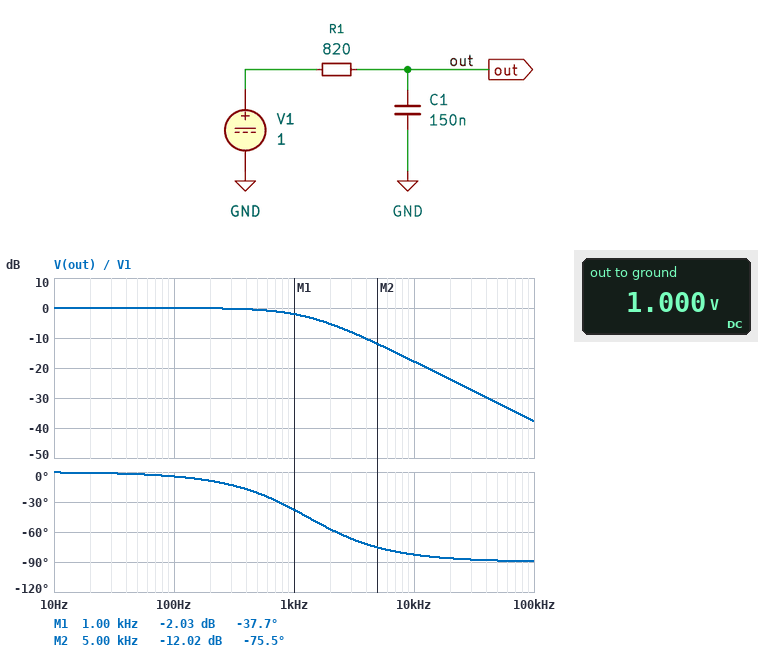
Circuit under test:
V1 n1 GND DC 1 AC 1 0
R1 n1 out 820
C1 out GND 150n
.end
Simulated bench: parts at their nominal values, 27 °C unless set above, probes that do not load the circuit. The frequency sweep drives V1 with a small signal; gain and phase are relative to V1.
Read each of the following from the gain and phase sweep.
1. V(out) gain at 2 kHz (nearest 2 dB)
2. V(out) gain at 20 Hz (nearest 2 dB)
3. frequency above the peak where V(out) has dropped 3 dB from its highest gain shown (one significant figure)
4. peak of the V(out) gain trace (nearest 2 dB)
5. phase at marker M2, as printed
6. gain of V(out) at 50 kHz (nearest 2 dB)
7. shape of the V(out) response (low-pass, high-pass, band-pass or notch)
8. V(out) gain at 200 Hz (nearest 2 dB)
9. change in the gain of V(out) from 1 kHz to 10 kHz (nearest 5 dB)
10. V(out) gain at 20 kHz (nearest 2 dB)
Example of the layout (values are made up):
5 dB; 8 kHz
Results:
-6 dB; 0 dB; 1 kHz; 0 dB; -75.5 deg; -32 dB; low-pass; 0 dB; -15 dB; -24 dB
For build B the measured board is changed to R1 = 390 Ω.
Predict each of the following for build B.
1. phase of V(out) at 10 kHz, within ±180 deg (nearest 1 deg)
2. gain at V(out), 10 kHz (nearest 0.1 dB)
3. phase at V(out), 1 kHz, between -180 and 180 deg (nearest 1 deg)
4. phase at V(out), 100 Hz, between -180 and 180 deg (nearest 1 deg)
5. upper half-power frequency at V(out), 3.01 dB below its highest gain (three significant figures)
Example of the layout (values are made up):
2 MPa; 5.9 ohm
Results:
-75 deg; -11.6 dB; -20 deg; -2 deg; 2.72 kHz
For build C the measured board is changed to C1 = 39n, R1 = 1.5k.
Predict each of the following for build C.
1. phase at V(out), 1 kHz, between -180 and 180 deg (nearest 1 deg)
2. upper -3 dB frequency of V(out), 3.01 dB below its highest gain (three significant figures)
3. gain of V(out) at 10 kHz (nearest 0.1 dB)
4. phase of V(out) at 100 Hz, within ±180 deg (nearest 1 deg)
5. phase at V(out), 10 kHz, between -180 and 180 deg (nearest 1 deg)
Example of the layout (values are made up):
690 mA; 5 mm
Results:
-20 deg; 2.72 kHz; -11.6 dB; -2 deg; -75 deg
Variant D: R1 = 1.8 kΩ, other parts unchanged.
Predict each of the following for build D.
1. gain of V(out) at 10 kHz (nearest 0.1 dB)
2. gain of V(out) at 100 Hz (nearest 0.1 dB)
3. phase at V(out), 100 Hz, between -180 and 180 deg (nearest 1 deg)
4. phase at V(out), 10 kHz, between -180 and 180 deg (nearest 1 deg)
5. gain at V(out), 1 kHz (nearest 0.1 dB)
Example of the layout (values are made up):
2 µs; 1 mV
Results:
-24.6 dB; -0.1 dB; -10 deg; -87 deg; -5.9 dB
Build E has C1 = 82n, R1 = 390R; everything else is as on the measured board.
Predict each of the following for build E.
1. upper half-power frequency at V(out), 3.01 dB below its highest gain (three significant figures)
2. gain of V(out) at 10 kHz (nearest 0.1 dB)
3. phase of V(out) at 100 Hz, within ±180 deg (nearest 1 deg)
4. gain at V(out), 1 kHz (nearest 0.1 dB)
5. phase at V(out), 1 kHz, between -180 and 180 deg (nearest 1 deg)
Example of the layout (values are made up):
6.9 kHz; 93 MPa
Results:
4.98 kHz; -7.0 dB; -1 deg; -0.2 dB; -11 deg
